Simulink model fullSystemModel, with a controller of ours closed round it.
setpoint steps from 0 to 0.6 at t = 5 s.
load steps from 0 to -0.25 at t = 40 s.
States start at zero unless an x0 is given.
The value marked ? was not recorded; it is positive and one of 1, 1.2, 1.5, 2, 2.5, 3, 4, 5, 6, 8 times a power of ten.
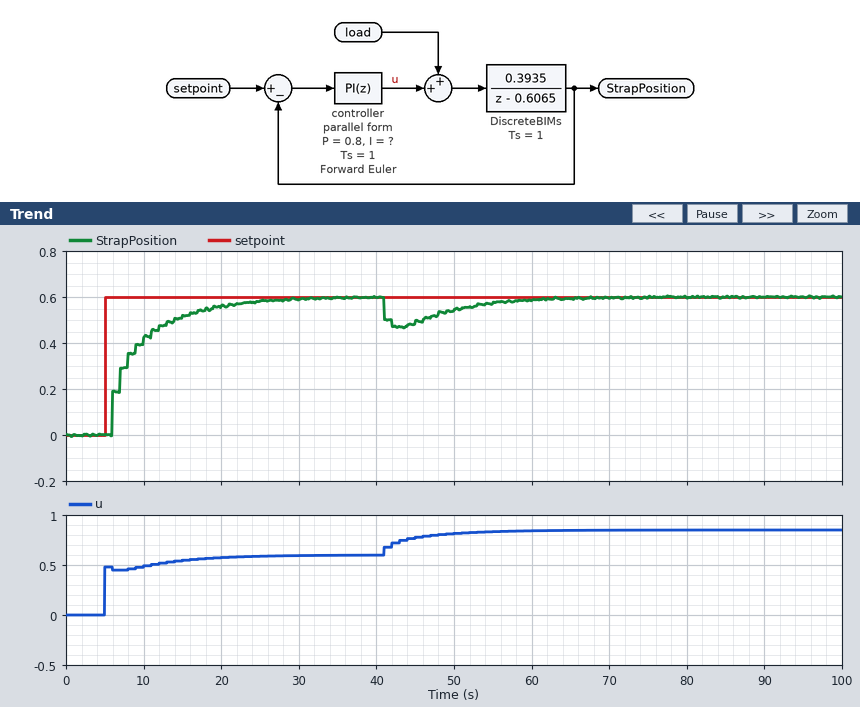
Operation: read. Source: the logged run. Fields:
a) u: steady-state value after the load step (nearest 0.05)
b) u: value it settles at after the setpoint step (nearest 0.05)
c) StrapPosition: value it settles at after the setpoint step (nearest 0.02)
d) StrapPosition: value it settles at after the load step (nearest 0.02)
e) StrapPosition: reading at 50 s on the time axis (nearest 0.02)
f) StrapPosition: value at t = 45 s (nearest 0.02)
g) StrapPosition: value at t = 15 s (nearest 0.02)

0.85
0.60
0.60
0.60
0.54
0.50
0.52
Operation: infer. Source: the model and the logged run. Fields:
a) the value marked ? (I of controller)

0.2
